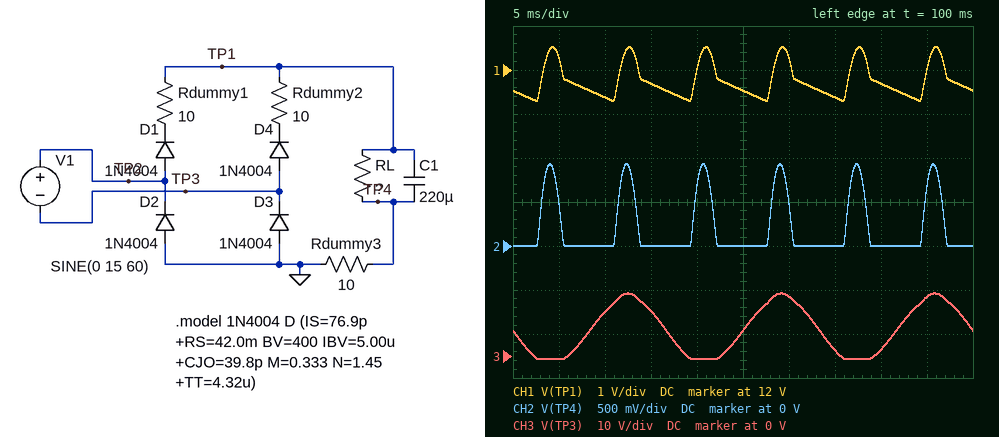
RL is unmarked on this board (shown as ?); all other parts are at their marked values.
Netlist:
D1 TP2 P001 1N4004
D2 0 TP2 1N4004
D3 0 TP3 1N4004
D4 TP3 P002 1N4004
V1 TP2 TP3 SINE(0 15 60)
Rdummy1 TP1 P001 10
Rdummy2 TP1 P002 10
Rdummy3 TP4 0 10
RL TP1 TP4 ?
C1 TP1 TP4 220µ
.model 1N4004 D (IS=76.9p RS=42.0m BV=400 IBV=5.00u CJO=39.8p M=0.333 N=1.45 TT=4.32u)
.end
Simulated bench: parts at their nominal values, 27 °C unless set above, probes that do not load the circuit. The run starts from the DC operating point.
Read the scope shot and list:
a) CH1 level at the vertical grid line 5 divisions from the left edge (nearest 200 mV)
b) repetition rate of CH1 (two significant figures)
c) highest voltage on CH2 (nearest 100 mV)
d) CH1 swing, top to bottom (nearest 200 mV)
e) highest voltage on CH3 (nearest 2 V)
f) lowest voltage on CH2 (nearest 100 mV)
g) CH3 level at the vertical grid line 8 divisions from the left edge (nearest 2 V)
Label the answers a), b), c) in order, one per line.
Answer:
a) 11.6 V
b) 120 Hz
c) 900 mV
d) 1.2 V
e) 14 V
f) 0 V
g) 2 V
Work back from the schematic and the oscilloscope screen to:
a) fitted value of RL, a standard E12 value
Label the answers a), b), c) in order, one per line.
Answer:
a) 560 Ω
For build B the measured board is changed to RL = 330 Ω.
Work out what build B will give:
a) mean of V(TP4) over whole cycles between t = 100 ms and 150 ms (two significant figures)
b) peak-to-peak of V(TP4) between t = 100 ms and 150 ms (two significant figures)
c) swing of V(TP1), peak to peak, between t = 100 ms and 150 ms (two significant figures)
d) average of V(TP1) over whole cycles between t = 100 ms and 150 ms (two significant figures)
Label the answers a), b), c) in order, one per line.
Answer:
a) 330 mV
b) 1.3 V
c) 1.7 V
d) 11 V
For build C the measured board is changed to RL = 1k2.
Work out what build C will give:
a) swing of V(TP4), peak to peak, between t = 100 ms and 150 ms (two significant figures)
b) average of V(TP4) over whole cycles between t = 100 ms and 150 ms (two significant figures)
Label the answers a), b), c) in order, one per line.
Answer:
a) 580 mV
b) 100 mV
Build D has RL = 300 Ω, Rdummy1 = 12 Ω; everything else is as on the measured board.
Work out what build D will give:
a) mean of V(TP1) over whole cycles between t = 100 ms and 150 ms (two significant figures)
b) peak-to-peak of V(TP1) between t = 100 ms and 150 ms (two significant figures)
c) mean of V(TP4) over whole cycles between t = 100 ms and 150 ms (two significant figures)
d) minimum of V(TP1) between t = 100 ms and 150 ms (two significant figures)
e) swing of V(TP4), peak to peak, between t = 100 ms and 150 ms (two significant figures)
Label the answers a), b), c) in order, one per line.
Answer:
a) 11 V
b) 1.9 V
c) 350 mV
d) 10 V
e) 1.4 V
